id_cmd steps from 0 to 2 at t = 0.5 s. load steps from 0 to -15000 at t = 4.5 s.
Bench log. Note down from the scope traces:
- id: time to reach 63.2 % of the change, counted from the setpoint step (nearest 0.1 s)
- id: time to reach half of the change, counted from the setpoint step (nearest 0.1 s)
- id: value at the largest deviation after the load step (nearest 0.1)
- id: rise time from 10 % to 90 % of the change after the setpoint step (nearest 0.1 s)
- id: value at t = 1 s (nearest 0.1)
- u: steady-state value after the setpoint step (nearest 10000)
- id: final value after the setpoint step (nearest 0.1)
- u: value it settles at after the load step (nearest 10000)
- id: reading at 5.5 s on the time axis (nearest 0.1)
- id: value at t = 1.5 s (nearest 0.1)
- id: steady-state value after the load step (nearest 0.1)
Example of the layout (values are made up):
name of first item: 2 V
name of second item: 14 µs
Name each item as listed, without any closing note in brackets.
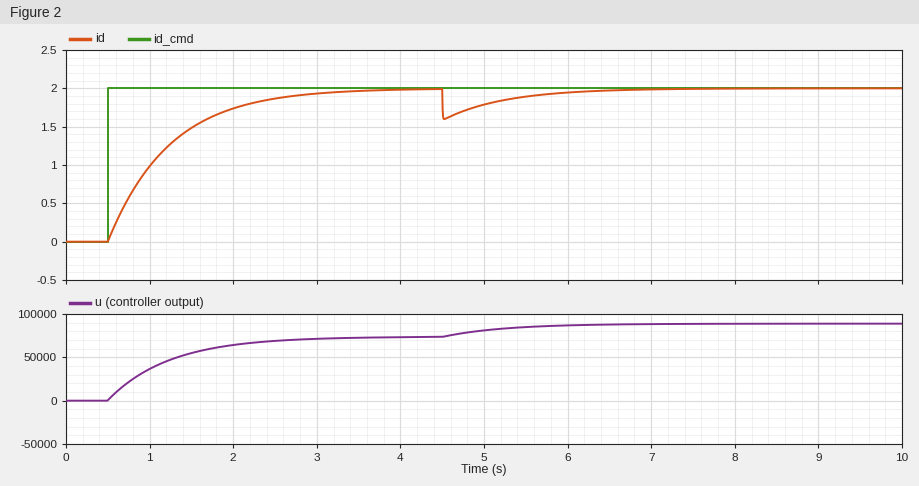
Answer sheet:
id: time to reach 63.2 % of the change, counted from the setpoint step: 0.7 s
id: time to reach half of the change, counted from the setpoint step: 0.5 s
id: value at the largest deviation after the load step: 1.6
id: rise time from 10 % to 90 % of the change after the setpoint step: 1.6 s
id: value at t = 1 s: 1.0
u: steady-state value after the setpoint step: 70000
id: final value after the setpoint step: 2.0
u: value it settles at after the load step: 90000
id: reading at 5.5 s on the time axis: 1.9
id: value at t = 1.5 s: 1.5
id: steady-state value after the load step: 2.0
